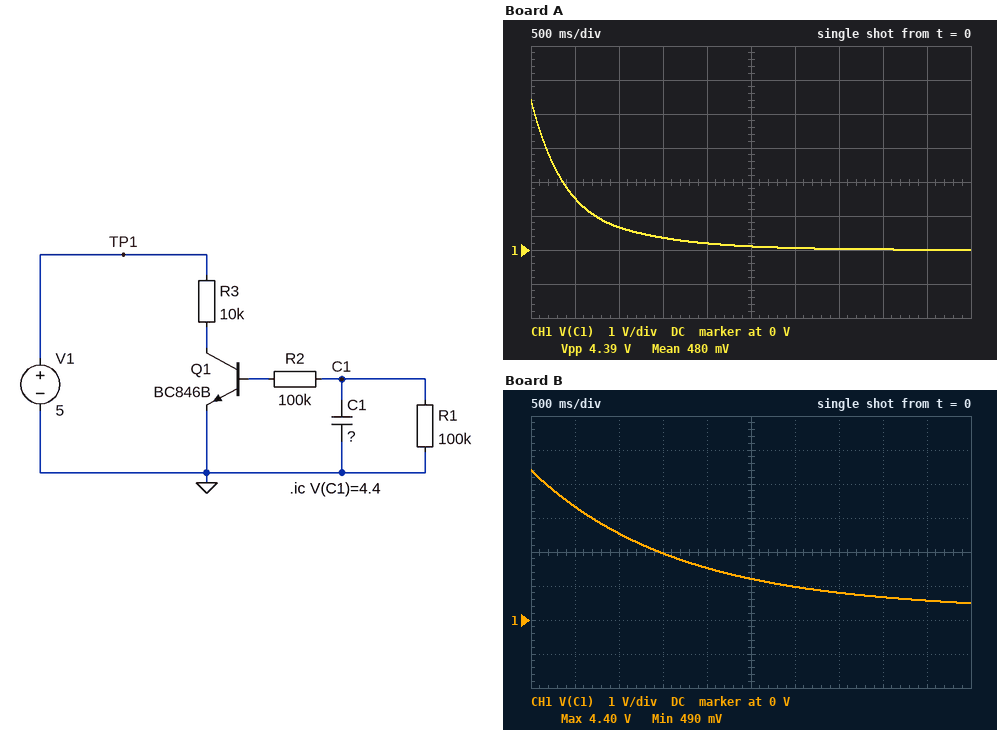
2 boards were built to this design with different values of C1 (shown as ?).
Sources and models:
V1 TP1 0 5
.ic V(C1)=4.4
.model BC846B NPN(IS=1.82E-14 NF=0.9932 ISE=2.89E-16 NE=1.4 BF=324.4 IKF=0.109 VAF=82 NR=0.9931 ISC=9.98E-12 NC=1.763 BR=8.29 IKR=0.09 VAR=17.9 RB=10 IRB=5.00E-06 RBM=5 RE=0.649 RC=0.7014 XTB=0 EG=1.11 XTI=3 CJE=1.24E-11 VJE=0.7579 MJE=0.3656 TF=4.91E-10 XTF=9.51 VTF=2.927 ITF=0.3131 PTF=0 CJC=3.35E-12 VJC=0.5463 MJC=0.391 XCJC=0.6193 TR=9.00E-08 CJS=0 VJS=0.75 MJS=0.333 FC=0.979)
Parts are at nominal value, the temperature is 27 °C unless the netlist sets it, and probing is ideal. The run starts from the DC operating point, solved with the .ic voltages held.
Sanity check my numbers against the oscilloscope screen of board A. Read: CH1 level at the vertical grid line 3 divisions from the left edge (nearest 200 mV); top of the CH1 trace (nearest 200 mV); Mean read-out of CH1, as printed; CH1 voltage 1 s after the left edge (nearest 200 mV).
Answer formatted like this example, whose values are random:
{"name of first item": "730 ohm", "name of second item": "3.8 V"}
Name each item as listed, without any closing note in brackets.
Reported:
{"CH1 level at the vertical grid line 3 divisions from the left edge": "400 mV", "top of the CH1 trace": "4.4 V", "Mean read-out of CH1, as printed": "480 mV", "CH1 voltage 1 s after the left edge": "600 mV"}
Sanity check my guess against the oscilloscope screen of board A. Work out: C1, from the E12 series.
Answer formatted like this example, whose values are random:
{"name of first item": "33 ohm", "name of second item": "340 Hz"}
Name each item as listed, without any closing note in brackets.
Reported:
{"C1, from the E12 series": "8.2 µF"}
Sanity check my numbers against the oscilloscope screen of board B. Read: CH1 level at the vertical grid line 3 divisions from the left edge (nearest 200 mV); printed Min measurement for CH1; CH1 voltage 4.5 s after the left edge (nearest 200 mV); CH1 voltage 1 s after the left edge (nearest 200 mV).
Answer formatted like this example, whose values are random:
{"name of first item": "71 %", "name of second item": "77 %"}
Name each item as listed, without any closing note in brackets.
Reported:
{"CH1 level at the vertical grid line 3 divisions from the left edge": "2.0 V", "printed Min measurement for CH1": "490 mV", "CH1 voltage 4.5 s after the left edge": "600 mV", "CH1 voltage 1 s after the left edge": "2.6 V"}
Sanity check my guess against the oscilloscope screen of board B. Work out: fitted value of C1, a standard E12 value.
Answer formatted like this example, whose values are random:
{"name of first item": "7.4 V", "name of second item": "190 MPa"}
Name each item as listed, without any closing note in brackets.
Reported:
{"fitted value of C1, a standard E12 value": "33 µF"}
